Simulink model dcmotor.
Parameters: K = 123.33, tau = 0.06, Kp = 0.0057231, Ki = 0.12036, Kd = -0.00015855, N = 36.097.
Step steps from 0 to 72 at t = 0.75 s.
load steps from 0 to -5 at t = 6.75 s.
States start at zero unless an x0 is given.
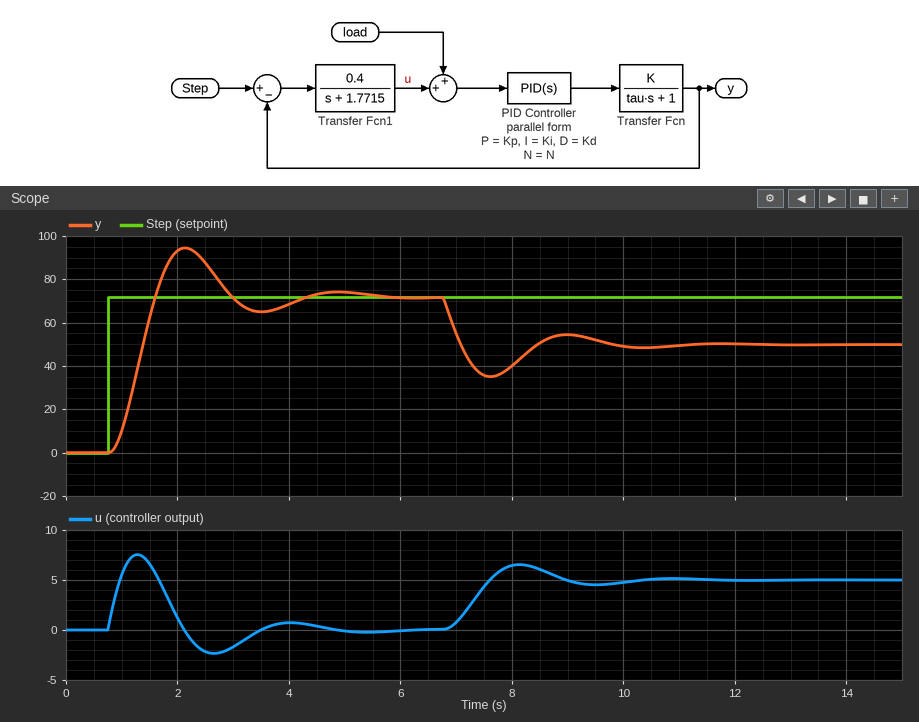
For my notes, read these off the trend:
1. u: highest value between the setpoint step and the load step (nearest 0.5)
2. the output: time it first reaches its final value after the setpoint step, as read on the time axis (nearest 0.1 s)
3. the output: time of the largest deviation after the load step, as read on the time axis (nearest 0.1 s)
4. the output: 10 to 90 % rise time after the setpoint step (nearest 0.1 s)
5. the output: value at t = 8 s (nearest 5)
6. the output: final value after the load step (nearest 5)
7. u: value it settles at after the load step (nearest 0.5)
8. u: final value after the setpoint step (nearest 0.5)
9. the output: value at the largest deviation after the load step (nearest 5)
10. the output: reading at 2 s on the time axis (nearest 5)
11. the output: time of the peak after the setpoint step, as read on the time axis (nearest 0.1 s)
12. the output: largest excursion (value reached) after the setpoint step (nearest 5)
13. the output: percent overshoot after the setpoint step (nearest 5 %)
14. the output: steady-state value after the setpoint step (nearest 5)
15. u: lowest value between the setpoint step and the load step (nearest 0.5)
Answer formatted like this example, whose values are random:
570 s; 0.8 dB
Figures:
7.5; 1.6 s; 7.6 s; 0.6 s; 40; 50; 5.0; 0.0; 35; 95; 2.1 s; 95; 30 %; 70; -2.5
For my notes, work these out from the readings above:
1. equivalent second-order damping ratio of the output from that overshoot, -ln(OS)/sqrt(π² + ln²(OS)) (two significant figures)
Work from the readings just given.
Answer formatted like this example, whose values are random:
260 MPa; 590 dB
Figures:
0.36
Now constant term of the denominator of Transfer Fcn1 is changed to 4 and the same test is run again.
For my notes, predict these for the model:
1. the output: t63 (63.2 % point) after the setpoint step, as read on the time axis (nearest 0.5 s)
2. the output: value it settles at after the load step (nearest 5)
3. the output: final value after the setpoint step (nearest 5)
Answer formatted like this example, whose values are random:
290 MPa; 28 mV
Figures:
1.5 s; 20; 70
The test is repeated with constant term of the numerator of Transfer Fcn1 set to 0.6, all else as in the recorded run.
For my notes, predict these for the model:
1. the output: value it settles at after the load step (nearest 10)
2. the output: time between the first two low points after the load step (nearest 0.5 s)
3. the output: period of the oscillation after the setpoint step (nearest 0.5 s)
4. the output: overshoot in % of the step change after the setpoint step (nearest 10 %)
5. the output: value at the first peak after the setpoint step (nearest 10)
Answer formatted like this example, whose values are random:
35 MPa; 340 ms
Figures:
60; 2.0 s; 2.0 s; 40 %; 100
